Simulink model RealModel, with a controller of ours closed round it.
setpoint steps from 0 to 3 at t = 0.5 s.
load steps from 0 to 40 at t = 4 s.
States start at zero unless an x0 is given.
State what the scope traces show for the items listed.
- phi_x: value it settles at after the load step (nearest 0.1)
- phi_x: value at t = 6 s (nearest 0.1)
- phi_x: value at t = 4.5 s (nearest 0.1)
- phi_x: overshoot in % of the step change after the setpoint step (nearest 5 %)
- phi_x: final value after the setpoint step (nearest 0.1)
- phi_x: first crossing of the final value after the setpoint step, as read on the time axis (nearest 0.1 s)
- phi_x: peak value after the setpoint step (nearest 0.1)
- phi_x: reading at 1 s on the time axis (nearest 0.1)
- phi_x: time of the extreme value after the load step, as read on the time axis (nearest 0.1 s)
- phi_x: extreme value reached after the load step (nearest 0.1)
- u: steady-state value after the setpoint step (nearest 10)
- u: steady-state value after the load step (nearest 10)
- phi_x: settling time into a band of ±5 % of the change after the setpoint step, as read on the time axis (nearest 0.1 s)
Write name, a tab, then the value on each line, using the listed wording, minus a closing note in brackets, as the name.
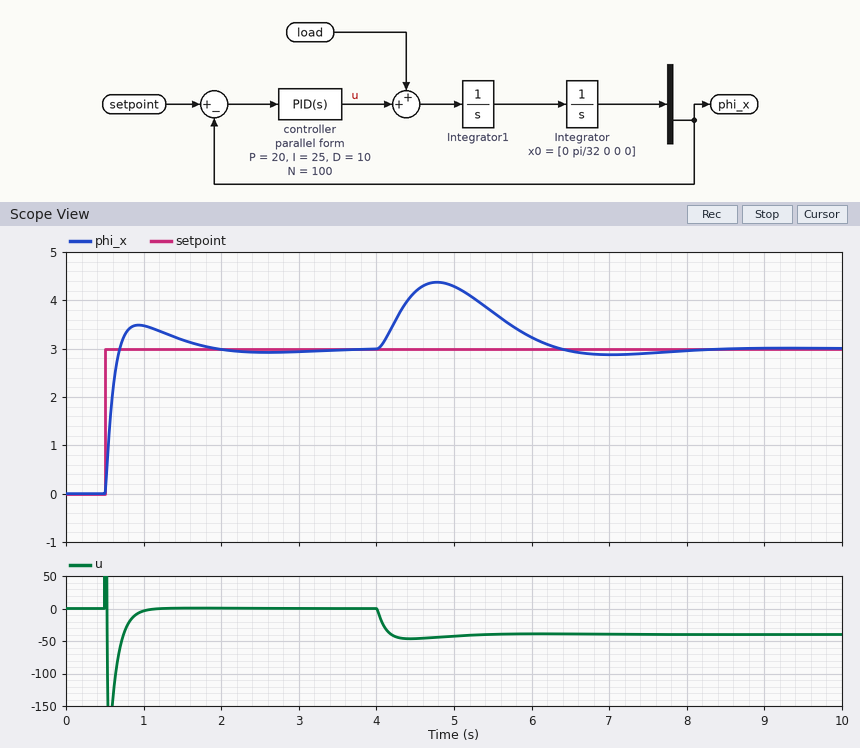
phi_x: value it settles at after the load step	3.0
phi_x: value at t = 6 s	3.2
phi_x: value at t = 4.5 s	4.2
phi_x: overshoot in % of the step change after the setpoint step	15 %
phi_x: final value after the setpoint step	3.0
phi_x: first crossing of the final value after the setpoint step, as read on the time axis	0.7 s
phi_x: peak value after the setpoint step	3.5
phi_x: reading at 1 s on the time axis	3.5
phi_x: time of the extreme value after the load step, as read on the time axis	4.8 s
phi_x: extreme value reached after the load step	4.4
u: steady-state value after the setpoint step	0
u: steady-state value after the load step	-40
phi_x: settling time into a band of ±5 % of the change after the setpoint step, as read on the time axis	1.6 s
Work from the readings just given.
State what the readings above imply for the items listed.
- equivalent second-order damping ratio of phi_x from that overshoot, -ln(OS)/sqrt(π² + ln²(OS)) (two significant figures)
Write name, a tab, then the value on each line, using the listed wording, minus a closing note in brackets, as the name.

equivalent second-order damping ratio of phi_x from that overshoot, -ln(OS)/sqrt(π² + ln²(OS))	0.52
